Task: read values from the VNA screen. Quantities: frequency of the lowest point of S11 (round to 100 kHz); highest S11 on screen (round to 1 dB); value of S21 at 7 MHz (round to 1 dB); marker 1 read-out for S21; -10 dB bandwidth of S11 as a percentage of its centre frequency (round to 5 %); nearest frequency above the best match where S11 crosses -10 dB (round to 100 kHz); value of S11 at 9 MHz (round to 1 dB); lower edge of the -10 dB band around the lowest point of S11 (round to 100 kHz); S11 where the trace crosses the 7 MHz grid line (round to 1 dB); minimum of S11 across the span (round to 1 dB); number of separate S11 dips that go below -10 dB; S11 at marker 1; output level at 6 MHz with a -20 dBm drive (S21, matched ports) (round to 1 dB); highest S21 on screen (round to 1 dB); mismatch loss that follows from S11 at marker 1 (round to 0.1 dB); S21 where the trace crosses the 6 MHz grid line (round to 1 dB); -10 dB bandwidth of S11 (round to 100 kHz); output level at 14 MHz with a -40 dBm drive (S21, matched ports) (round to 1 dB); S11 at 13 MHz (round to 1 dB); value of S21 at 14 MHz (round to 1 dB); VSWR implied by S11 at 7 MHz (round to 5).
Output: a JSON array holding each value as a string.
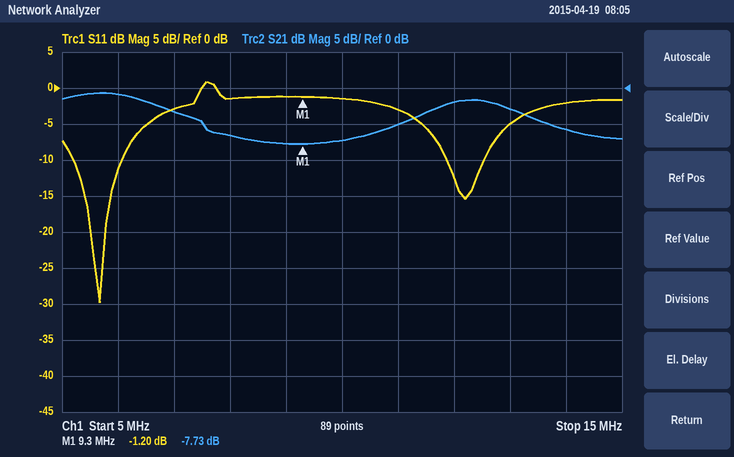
["5.7 MHz", "1 dB", "-3 dB", "-7.73 dB", "15 %", "6.1 MHz", "-1 dB", "5.2 MHz", "-3 dB", "-30 dB", "2", "-1.20 dB", "-21 dBm", "-1 dB", "6.2 dB", "-1 dB", "900 kHz", "-46 dBm", "-5 dB", "-6 dB", "5"]
